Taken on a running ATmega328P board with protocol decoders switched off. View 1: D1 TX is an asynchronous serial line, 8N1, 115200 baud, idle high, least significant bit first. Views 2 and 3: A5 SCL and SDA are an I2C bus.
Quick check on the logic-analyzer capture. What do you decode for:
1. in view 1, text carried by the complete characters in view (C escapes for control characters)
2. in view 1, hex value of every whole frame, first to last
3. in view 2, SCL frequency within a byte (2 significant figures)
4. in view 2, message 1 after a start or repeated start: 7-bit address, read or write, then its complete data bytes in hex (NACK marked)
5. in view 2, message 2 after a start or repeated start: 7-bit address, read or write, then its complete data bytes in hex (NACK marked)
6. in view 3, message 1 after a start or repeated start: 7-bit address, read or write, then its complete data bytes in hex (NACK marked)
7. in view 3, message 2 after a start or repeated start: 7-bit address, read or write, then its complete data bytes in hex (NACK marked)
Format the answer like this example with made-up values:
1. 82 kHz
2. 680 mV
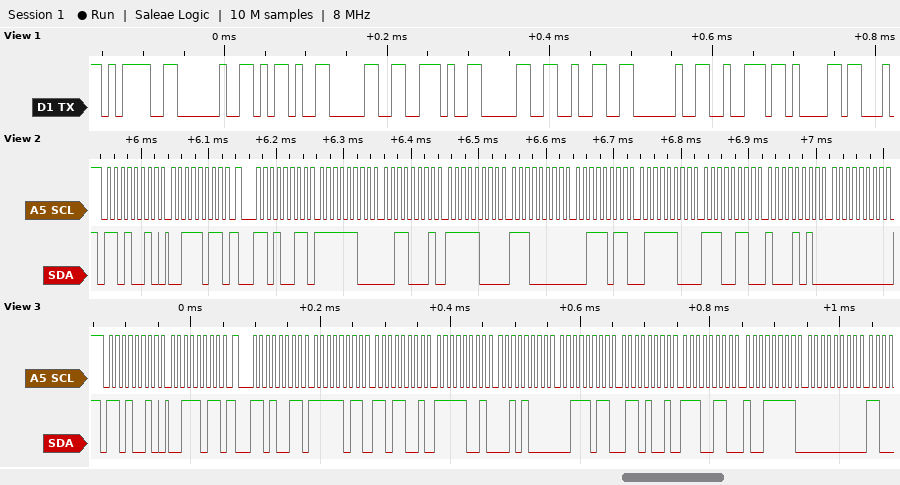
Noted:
1. "= -0.02 ra"
2. 0x3D 0x20 0x2D 0x30 0x2E 0x30 0x32 0x20 0x72 0x61
3. 100 kHz
4. 0x69 write: 3B
5. 0x69 read: FC 31 F8 E0 3B 7C E6 8A 00
6. 0x69 write: 3B
7. 0x69 read: FB D9 F9 28 3B 69 E6 9F 00
